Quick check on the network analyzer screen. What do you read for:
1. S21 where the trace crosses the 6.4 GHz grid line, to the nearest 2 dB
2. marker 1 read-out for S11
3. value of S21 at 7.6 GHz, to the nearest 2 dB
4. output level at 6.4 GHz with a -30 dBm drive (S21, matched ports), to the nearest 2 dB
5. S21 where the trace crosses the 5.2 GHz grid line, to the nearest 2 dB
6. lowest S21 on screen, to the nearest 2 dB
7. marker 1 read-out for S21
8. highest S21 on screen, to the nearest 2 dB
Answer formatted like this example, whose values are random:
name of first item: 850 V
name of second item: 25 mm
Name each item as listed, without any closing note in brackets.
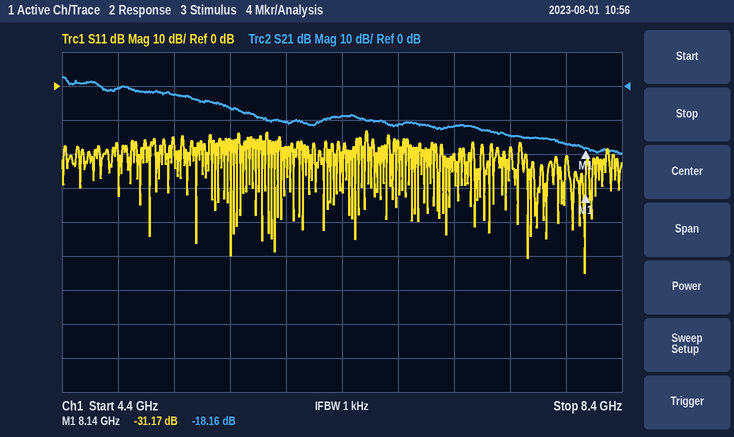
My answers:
S21 where the trace crosses the 6.4 GHz grid line, to the nearest 2 dB: -8 dB
marker 1 read-out for S11: -31.17 dB
value of S21 at 7.6 GHz, to the nearest 2 dB: -14 dB
output level at 6.4 GHz with a -30 dBm drive (S21, matched ports), to the nearest 2 dB: -38 dBm
S21 where the trace crosses the 5.2 GHz grid line, to the nearest 2 dB: -2 dB
lowest S21 on screen, to the nearest 2 dB: -20 dB
marker 1 read-out for S21: -18.16 dB
highest S21 on screen, to the nearest 2 dB: 2 dB
